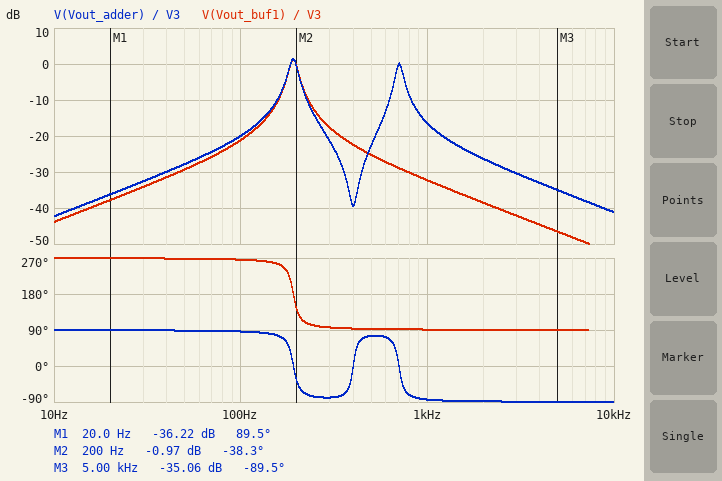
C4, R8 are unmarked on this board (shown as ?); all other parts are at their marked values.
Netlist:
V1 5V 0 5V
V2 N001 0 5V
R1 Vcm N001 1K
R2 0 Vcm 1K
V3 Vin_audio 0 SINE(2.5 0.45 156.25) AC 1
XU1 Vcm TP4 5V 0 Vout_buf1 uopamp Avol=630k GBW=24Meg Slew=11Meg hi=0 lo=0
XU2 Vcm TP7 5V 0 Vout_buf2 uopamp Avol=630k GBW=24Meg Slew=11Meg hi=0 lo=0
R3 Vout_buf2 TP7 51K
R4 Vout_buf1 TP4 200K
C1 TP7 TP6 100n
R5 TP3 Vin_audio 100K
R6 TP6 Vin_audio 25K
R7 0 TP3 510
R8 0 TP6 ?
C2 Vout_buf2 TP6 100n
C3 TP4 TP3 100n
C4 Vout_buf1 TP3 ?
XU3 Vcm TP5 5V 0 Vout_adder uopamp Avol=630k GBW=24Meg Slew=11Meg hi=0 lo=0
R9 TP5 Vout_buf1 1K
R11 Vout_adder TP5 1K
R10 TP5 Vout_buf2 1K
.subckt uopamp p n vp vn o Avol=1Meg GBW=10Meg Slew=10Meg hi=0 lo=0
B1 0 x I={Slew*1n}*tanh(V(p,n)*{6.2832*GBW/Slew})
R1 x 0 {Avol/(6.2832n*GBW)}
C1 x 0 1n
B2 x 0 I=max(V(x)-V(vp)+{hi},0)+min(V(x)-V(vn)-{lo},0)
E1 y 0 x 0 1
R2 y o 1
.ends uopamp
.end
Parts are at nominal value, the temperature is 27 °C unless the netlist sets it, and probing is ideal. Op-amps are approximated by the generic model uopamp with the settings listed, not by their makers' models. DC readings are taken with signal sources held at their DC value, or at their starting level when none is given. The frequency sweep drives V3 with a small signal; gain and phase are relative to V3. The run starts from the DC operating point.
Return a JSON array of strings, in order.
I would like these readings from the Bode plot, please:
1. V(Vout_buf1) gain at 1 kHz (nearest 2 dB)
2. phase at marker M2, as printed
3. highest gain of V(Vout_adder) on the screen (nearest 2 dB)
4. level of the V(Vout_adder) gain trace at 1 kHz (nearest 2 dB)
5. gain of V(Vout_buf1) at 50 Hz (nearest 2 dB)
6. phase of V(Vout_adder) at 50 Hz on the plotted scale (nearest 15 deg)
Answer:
["-32 dB", "-38.3 deg", "2 dB", "-16 dB", "-30 dB", "90 deg"]
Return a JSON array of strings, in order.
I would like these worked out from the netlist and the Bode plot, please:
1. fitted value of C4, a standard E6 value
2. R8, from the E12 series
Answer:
["68 nF", "100 Ω"]
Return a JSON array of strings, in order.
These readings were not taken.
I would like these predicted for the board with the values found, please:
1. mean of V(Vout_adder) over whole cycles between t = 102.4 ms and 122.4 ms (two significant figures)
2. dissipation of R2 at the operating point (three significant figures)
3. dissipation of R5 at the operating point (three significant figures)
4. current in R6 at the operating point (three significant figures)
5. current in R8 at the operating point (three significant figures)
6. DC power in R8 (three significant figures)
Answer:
["2.5 V", "6.25 mW", "61.9 µW", "99.6 µA", "99.6 µA", "992 nW"]
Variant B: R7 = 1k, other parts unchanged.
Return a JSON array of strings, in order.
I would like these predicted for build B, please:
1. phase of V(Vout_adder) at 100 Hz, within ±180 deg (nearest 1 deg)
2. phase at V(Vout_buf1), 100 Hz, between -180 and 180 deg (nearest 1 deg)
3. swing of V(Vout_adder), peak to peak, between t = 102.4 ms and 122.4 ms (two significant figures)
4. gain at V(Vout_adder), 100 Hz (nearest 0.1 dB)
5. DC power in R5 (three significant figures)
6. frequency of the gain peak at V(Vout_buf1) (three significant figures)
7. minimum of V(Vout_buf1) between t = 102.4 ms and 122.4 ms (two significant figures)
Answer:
["78 deg", "-103 deg", "500 mV", "-11.3 dB", "61.3 µW", "137 Hz", "2.2 V"]
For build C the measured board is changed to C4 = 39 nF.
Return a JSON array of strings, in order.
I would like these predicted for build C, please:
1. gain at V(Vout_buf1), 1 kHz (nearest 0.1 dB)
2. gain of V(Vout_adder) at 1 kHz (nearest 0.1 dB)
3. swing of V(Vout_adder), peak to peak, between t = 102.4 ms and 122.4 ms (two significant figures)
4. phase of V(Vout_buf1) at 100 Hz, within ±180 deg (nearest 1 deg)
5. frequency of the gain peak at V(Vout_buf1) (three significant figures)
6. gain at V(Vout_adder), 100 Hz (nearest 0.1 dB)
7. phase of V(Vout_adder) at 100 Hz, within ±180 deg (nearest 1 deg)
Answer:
["-27.2 dB", "-15.4 dB", "160 mV", "-93 deg", "253 Hz", "-21.1 dB", "87 deg"]
